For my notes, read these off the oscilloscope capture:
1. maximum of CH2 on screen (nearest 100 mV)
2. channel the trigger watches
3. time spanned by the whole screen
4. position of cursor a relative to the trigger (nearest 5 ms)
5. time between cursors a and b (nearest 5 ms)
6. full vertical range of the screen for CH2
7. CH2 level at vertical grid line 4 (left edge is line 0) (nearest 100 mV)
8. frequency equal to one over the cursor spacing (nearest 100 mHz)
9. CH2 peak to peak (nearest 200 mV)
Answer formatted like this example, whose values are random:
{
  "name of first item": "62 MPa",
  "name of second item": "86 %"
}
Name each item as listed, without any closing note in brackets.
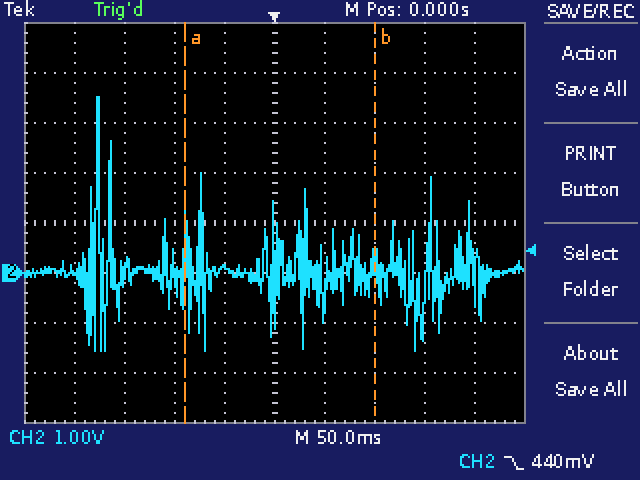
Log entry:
{
  "maximum of CH2 on screen": "3.5 V",
  "channel the trigger watches": "CH2",
  "time spanned by the whole screen": "500 ms",
  "position of cursor a relative to the trigger": "-90 ms",
  "time between cursors a and b": "190 ms",
  "full vertical range of the screen for CH2": "8 V",
  "CH2 level at vertical grid line 4 (left edge is line 0)": "100 mV",
  "frequency equal to one over the cursor spacing": "5.3 Hz",
  "CH2 peak to peak": "5.0 V"
}
